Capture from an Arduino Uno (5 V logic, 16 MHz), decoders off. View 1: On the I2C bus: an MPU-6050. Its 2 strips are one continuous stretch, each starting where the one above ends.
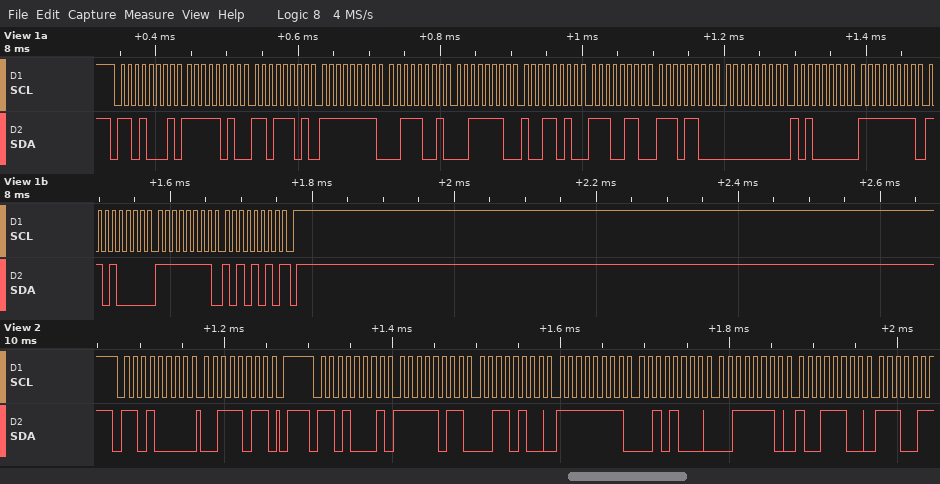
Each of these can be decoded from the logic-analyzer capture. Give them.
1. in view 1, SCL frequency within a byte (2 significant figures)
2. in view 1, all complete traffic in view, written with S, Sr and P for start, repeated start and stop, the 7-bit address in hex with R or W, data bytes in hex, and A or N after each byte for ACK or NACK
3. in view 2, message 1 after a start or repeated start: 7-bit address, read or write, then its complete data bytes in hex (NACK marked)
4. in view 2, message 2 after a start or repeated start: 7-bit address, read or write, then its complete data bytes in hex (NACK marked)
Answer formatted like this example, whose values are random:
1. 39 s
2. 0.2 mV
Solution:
1. 100 kHz
2. S 68R A FA A DD A FF A 39 A 3E A 9A A E6 A EC A 00 A A0 A FF A D0 A FF A AA N P
3. 0x68 write: 3B
4. 0x68 read: FB 34 FF 28 3E 9C
